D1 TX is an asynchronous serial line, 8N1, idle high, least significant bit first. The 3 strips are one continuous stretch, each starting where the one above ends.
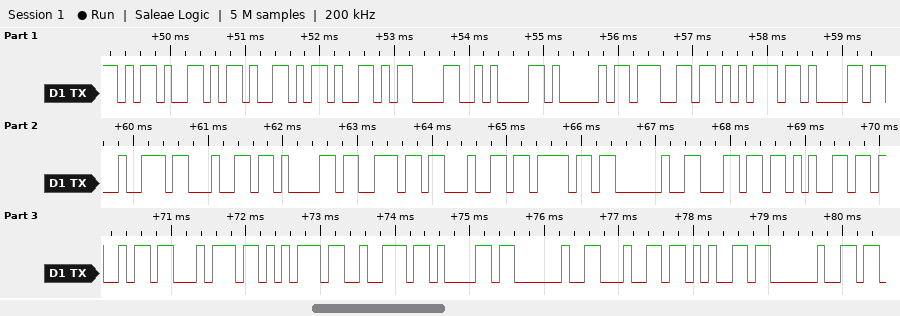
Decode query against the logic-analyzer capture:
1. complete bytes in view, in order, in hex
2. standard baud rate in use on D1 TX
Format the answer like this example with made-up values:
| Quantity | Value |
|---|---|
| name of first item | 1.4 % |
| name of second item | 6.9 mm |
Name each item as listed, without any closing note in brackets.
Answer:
| Quantity | Value |
|---|---|
| complete bytes in view, in order, in hex | 2D 2D 2D 0D 0A 41 67 75 61 72 64 61 6E 64 6F 20 6C 65 69 74 75 72 61 20 64 65 20 |
| standard baud rate in use on D1 TX | 9600 baud |
